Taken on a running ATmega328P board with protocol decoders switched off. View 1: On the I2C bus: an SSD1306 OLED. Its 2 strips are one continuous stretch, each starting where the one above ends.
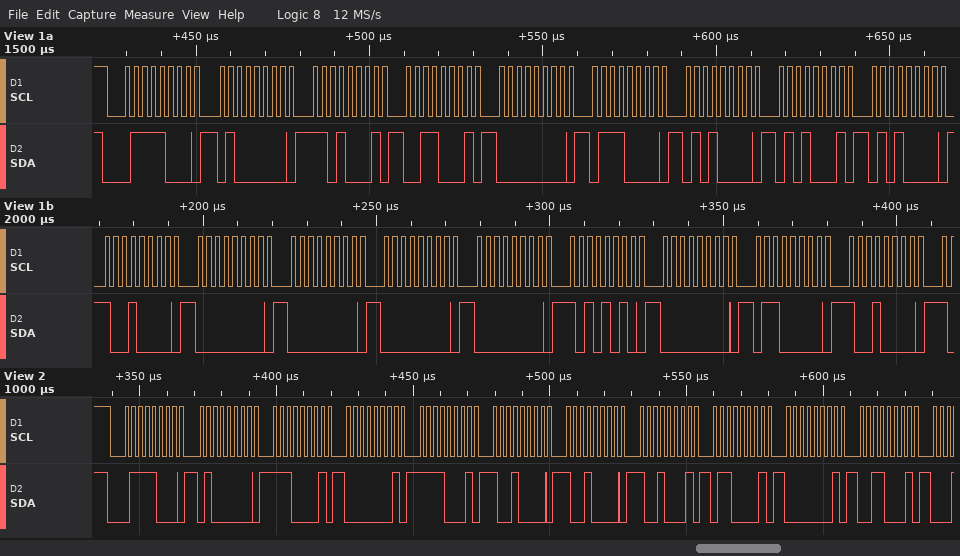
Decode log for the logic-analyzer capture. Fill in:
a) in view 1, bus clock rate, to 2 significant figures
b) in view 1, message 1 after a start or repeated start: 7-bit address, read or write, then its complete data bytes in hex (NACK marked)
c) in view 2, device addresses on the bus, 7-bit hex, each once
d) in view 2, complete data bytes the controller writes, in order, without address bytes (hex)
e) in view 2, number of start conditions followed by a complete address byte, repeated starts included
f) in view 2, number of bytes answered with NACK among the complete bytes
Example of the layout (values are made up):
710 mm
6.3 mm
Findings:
400 kHz
0x3C write: 40 D1 31 00 70 50 51 50 90 00 00 00 00 AA 00 60 90
0x3C
40 E1 01 F1 90 90 91 61 01 31
1
0
